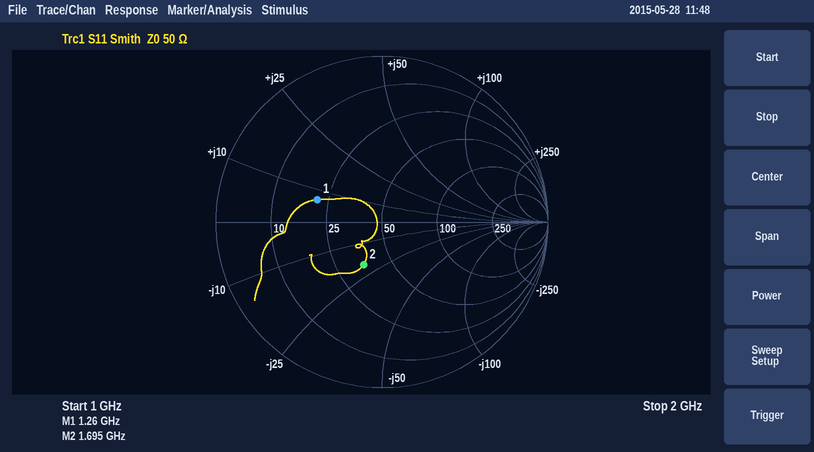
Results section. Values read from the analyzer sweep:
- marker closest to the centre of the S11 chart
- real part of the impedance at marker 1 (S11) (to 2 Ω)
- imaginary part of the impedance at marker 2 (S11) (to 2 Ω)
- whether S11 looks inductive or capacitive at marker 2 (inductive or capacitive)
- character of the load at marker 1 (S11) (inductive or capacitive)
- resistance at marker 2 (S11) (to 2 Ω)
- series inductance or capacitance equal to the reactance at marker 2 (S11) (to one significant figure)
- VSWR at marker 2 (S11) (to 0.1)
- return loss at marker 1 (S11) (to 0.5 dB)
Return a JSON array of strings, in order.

["marker 2", "22 Ω", "-20 Ω", "capacitive", "inductive", "36 Ω", "5 pF", "1.8", "7.5 dB"]
